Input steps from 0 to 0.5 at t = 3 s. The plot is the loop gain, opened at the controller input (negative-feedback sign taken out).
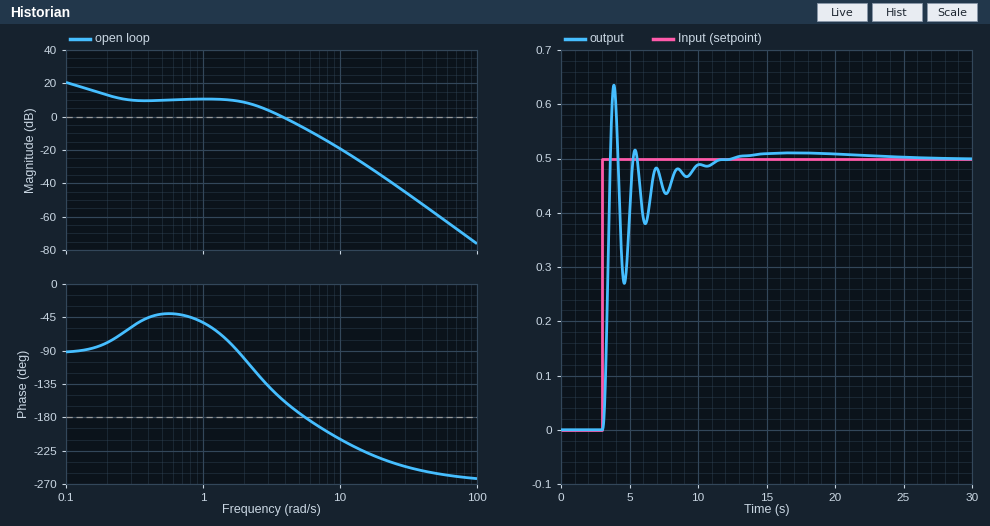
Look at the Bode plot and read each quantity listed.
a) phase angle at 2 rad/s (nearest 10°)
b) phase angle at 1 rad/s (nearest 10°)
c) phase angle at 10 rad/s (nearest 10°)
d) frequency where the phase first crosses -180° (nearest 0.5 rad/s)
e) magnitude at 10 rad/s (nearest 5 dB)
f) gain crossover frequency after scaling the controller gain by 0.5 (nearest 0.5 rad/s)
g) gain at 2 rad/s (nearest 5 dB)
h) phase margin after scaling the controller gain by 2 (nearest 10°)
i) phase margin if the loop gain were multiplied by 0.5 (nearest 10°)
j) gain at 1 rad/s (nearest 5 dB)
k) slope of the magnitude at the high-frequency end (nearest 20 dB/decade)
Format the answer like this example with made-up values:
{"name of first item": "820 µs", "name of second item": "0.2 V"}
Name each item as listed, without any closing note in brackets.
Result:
{"phase angle at 2 rad/s": "-100°", "phase angle at 1 rad/s": "-50°", "phase angle at 10 rad/s": "-210°", "frequency where the phase first crosses -180°": "5.5 rad/s", "magnitude at 10 rad/s": "-20 dB", "gain crossover frequency after scaling the controller gain by 0.5": "2.5 rad/s", "gain at 2 rad/s": "10 dB", "phase margin after scaling the controller gain by 2": "0°", "phase margin if the loop gain were multiplied by 0.5": "60°", "gain at 1 rad/s": "10 dB", "slope of the magnitude at the high-frequency end": "-60 dB/decade"}
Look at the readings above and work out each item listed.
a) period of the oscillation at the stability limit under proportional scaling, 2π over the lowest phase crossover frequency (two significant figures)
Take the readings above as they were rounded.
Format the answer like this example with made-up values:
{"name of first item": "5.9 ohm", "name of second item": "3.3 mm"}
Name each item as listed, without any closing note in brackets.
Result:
{"period of the oscillation at the stability limit under proportional scaling, 2π over the lowest phase crossover frequency": "1.1 s"}
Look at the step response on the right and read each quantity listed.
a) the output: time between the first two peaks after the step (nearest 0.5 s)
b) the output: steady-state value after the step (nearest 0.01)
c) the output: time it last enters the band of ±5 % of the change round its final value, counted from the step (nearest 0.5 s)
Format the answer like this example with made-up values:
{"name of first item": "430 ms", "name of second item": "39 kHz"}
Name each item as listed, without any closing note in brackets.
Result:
{"the output: time between the first two peaks after the step": "1.5 s", "the output: steady-state value after the step": "0.50", "the output: time it last enters the band of ±5 % of the change round its final value, counted from the step": "6.5 s"}
